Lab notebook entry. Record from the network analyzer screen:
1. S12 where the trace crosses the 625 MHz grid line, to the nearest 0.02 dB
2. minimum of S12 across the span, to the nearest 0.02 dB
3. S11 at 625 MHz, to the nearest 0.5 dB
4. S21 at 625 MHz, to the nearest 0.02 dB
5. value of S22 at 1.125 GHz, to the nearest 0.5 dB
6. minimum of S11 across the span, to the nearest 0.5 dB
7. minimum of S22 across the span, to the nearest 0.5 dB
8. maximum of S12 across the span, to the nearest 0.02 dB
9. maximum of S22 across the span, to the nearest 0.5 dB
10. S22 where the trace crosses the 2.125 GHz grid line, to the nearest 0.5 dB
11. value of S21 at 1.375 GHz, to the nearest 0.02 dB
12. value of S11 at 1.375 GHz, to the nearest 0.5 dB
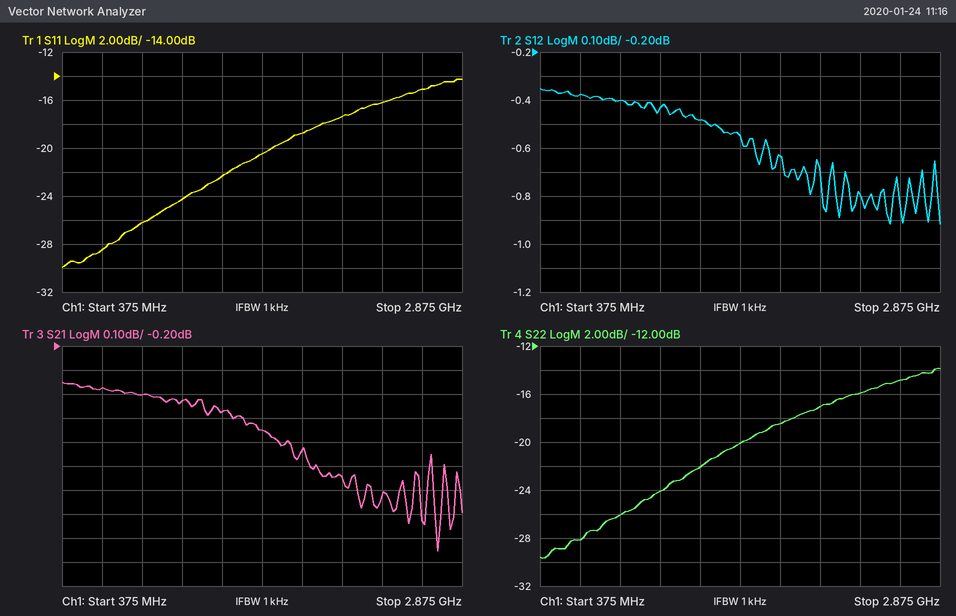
-0.38 dB
-0.92 dB
-28.5 dB
-0.38 dB
-24.0 dB
-30.0 dB
-29.5 dB
-0.36 dB
-14.0 dB
-17.0 dB
-0.48 dB
-22.5 dB
